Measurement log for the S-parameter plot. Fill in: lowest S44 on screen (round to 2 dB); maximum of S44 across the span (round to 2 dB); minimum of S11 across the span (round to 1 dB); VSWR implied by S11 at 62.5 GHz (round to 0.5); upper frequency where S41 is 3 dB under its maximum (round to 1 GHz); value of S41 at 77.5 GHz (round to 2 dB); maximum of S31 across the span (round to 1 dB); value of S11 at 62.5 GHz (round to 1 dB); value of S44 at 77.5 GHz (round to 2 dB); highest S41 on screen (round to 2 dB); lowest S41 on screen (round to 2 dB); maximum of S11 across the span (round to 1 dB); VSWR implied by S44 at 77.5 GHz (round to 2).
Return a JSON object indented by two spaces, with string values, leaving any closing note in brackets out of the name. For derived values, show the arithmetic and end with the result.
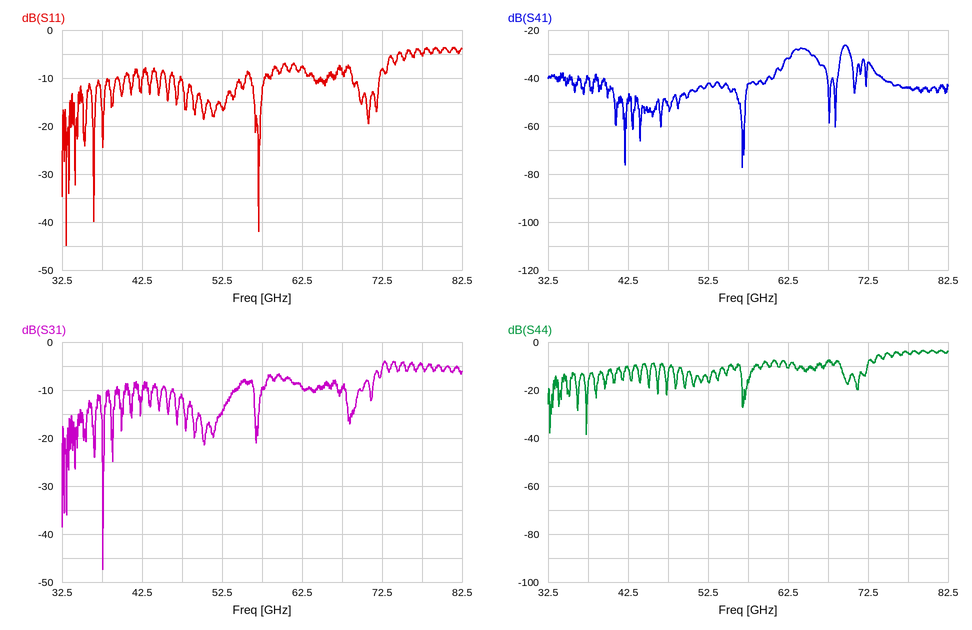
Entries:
{
  "lowest S44 on screen": "-38 dB",
  "maximum of S44 across the span": "-4 dB",
  "minimum of S11 across the span": "-45 dB",
  "VSWR implied by S11 at 62.5 GHz": "|Γ| = 10^(-8/20) = 0.3981; VSWR = (1 + 0.3981)/(1 − 0.3981) ≈ 2.32, so 2.5 to the nearest 0.5",
  "upper frequency where S41 is 3 dB under its maximum": "70 GHz",
  "value of S41 at 77.5 GHz": "-44 dB",
  "maximum of S31 across the span": "-4 dB",
  "value of S11 at 62.5 GHz": "-8 dB",
  "value of S44 at 77.5 GHz": "-4 dB",
  "highest S41 on screen": "-26 dB",
  "lowest S41 on screen": "-78 dB",
  "maximum of S11 across the span": "-4 dB",
  "VSWR implied by S44 at 77.5 GHz": "|Γ| = 10^(-4/20) = 0.6310; VSWR = (1 + 0.6310)/(1 − 0.6310) ≈ 4"
}
